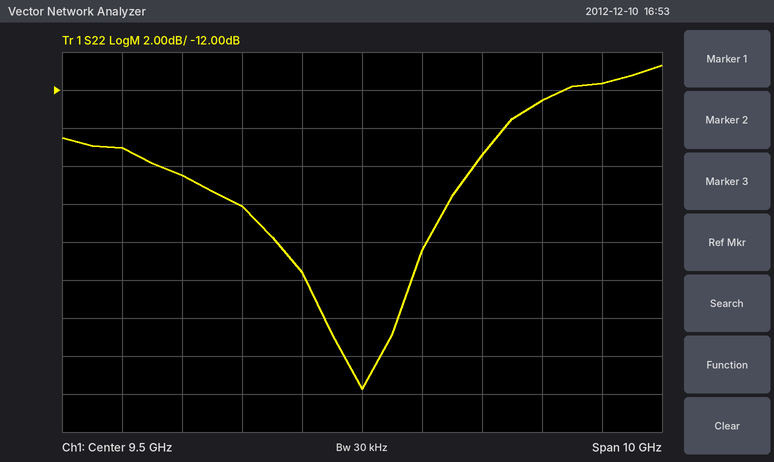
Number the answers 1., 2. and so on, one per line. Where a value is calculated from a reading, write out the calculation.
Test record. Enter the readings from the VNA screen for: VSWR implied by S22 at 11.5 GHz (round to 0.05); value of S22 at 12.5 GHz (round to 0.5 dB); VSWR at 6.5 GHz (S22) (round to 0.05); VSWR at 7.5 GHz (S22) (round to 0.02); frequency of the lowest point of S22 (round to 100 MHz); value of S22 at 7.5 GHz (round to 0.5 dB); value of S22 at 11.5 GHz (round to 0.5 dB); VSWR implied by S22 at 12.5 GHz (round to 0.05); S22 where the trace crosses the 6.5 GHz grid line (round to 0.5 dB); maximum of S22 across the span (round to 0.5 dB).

1. |Γ| = 10^(-15.5/20) = 0.1679; VSWR = (1 + 0.1679)/(1 − 0.1679) ≈ 1.40
2. -12.5 dB
3. |Γ| = 10^(-16.5/20) = 0.1496; VSWR = (1 + 0.1496)/(1 − 0.1496) ≈ 1.35
4. |Γ| = 10^(-18/20) = 0.1259; VSWR = (1 + 0.1259)/(1 − 0.1259) ≈ 1.29, so 1.28 to the nearest 0.02
5. 9.5 GHz
6. -18.0 dB
7. -15.5 dB
8. |Γ| = 10^(-12.5/20) = 0.2371; VSWR = (1 + 0.2371)/(1 − 0.2371) ≈ 1.62, so 1.60 to the nearest 0.05
9. -16.5 dB
10. -10.5 dB
